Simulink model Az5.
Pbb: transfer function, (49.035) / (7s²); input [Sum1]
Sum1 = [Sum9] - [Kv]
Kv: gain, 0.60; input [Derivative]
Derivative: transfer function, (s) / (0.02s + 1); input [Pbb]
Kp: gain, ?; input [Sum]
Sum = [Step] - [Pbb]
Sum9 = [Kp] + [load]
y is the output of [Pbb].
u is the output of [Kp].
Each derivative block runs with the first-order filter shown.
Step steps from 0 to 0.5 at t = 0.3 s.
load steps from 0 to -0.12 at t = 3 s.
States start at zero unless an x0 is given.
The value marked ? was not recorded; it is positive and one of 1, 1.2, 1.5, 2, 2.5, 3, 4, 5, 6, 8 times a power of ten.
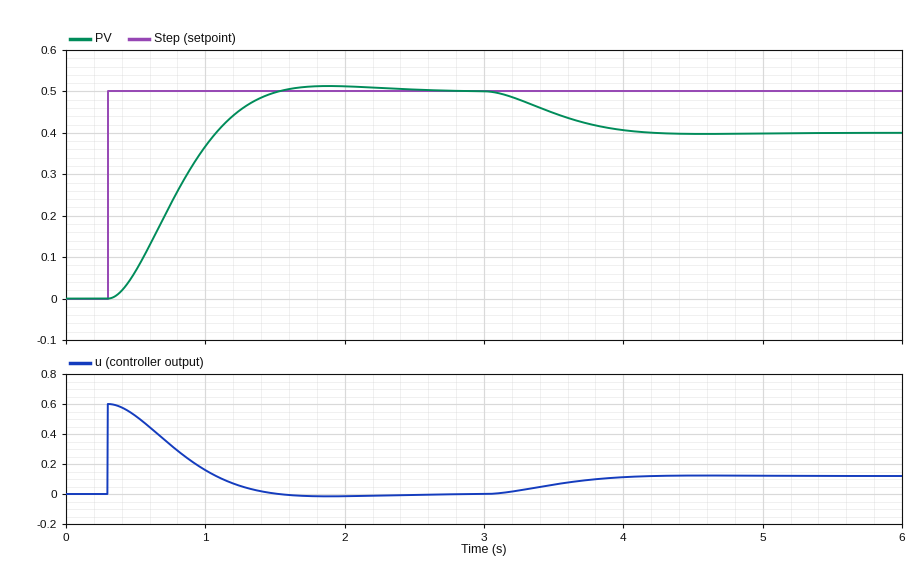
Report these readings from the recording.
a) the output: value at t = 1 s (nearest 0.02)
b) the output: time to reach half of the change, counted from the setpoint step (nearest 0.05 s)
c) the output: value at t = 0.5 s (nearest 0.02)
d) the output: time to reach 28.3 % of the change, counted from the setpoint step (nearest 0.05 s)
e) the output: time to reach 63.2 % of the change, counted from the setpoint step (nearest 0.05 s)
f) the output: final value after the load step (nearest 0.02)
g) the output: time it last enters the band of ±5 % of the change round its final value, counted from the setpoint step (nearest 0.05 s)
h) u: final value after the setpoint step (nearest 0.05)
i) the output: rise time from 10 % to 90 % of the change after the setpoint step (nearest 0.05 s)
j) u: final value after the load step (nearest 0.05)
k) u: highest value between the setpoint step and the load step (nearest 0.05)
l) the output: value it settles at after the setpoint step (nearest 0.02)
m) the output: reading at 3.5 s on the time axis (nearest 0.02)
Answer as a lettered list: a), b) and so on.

a) 0.36
b) 0.50 s
c) 0.06
d) 0.30 s
e) 0.60 s
f) 0.40
g) 1.05 s
h) 0.00
i) 0.75 s
j) 0.10
k) 0.60
l) 0.50
m) 0.44
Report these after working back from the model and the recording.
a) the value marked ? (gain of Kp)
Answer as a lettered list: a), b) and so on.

a) 1.2
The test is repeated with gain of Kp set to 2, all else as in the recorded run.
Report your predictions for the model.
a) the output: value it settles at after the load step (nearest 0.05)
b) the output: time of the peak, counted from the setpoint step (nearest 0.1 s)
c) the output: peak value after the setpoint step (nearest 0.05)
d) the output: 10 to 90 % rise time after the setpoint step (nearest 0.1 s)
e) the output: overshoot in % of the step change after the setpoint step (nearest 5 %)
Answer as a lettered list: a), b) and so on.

a) 0.45
b) 1.0 s
c) 0.55
d) 0.5 s
e) 10 %
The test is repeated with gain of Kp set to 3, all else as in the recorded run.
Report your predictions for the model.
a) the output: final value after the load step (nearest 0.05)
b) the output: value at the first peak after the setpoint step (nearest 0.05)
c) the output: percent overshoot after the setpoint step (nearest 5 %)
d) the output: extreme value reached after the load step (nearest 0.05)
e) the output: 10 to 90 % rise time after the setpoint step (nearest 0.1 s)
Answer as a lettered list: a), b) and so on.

a) 0.45
b) 0.60
c) 20 %
d) 0.45
e) 0.3 s
